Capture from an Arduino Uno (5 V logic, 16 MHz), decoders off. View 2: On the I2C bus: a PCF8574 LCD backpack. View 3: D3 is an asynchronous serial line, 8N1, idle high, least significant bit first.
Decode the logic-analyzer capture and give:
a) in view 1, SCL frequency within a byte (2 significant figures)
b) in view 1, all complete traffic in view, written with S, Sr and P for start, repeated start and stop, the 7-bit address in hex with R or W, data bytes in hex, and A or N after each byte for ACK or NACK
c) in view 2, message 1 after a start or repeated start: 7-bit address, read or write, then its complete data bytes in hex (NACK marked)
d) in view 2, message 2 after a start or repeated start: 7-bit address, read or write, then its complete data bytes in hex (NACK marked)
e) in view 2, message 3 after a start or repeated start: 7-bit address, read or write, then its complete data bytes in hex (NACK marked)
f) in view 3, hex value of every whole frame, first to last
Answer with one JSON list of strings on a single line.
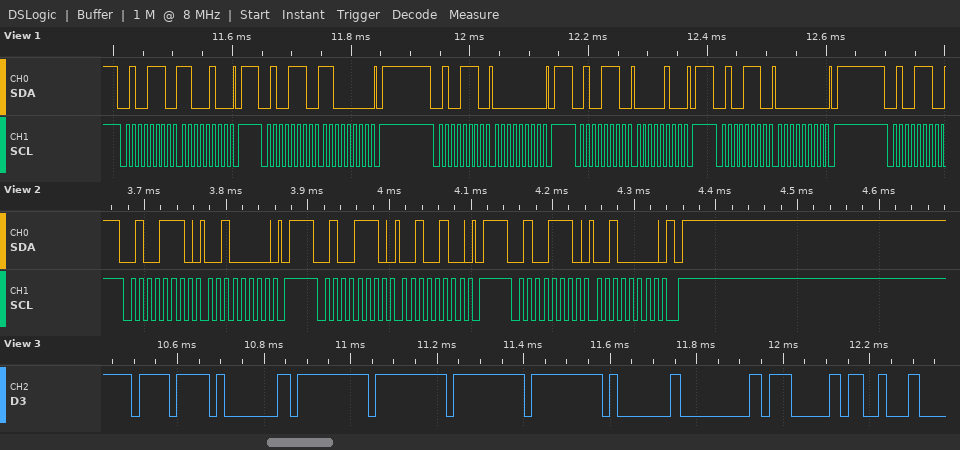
["100 kHz", "S 27W A C4 A P S 27W A C0 A P S 27W A 00 A P S 27W A 04 A P S 27W A 00 A P S 27W A", "0x27 write: 20", "0x27 write: 24", "0x27 write: 20", "0xEF 0x01 0xFF 0xFF 0xFF 0xFF 0x01 0x00 0x07 0x13"]
